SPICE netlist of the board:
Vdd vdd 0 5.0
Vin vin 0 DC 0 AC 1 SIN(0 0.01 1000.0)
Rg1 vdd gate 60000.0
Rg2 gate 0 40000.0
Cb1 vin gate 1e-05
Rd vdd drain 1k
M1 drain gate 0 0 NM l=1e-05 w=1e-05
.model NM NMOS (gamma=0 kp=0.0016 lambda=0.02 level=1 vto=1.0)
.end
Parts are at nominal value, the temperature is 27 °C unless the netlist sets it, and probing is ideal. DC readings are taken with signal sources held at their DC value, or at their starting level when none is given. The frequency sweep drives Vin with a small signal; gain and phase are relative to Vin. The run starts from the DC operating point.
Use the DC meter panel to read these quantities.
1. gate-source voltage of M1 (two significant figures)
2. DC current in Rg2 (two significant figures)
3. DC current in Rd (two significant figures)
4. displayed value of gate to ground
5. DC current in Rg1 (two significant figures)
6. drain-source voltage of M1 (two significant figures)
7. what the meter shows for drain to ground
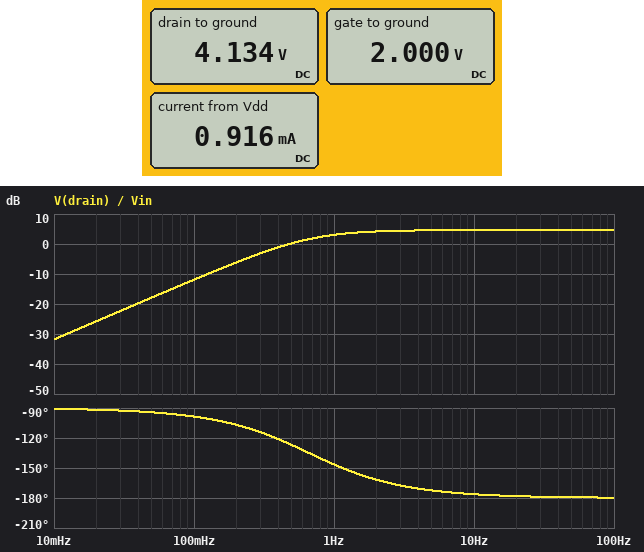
2.0 V
50 µA
870 µA
2.000 V
50 µA
4.1 V
4.134 V
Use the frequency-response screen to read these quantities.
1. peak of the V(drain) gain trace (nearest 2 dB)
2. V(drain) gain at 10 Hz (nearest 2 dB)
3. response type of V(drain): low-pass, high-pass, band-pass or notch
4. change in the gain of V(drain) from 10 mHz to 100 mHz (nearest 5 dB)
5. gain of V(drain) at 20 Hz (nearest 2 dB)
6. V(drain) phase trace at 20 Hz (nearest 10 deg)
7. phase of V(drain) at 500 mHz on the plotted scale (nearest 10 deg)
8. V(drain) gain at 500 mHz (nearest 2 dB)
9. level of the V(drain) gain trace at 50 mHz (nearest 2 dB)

4 dB
4 dB
high-pass
20 dB
4 dB
-180 deg
-130 deg
0 dB
-18 dB
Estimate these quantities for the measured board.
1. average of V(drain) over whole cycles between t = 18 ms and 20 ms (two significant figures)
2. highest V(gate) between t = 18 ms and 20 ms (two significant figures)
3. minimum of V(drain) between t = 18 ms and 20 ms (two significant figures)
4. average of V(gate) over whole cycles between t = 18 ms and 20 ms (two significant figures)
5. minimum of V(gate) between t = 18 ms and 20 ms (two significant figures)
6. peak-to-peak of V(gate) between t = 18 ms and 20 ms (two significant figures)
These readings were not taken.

4.1 V
2.0 V
4.1 V
2.0 V
2.0 V
20 mV
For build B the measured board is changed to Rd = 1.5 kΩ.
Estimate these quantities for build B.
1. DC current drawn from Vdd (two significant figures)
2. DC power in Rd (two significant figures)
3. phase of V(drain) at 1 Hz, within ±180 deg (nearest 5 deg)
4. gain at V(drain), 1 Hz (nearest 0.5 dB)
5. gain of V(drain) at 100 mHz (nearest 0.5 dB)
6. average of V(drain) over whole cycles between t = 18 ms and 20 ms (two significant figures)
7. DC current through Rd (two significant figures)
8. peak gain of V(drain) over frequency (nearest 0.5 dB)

910 µA
1.1 mW
-145 deg
6.5 dB
-8.5 dB
3.7 V
860 µA
8.0 dB
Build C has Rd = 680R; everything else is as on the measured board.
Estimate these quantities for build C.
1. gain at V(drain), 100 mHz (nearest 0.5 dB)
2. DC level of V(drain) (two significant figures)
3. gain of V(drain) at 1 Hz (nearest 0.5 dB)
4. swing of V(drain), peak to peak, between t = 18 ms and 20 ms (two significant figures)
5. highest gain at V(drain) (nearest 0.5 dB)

-15.0 dB
4.4 V
0 dB
23 mV
1.5 dB
